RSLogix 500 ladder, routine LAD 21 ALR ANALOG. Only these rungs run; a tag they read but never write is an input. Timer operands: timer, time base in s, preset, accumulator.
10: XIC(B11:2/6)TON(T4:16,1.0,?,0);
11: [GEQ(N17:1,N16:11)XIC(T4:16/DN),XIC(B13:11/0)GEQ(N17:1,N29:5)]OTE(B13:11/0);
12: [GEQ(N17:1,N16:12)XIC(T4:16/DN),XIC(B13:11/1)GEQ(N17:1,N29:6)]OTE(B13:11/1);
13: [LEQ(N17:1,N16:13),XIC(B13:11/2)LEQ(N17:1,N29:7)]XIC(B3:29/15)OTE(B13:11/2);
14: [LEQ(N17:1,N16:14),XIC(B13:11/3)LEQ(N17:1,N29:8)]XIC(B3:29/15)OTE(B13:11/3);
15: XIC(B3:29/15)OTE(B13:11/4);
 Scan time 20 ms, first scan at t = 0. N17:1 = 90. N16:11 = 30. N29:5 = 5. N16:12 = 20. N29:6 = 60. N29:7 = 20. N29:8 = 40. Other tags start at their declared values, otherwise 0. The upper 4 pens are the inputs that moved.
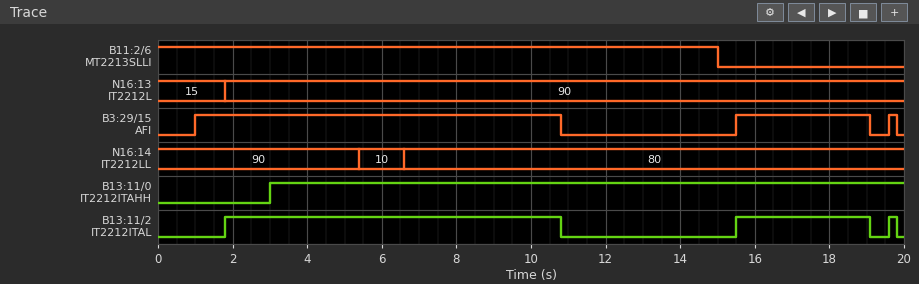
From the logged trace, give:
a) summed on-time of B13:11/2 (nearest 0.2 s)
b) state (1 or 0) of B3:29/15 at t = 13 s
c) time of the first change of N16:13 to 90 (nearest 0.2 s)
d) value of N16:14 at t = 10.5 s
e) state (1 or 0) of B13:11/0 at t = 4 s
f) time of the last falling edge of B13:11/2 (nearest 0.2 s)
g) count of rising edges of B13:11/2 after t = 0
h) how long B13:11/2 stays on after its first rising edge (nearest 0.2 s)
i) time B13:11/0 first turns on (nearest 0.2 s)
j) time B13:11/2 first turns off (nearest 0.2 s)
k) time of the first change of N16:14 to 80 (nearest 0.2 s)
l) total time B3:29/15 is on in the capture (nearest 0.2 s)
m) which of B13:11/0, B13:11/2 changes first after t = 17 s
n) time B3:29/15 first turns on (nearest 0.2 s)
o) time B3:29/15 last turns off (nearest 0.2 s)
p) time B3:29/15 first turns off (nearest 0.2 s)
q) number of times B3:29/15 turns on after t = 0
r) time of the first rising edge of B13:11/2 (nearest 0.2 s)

12.8 s
0
1.8 s
80
1
19.8 s
3
9.0 s
3.0 s
10.8 s
6.6 s
13.6 s
B13:11/2
1.0 s
19.8 s
10.8 s
3
1.8 s
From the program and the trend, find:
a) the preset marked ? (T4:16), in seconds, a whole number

3 s
